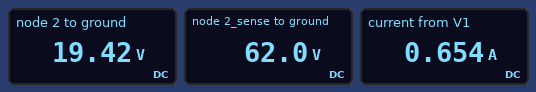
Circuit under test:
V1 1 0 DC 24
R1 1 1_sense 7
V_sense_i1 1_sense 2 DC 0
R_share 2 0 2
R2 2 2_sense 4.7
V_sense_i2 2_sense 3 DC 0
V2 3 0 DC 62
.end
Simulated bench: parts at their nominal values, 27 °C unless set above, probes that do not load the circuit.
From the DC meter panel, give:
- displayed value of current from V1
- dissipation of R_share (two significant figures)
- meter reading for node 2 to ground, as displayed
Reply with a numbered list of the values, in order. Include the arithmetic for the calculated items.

1. 0.654 A
2. (19.42 V)^2 / 2 Ω = 190 W
3. 19.42 V
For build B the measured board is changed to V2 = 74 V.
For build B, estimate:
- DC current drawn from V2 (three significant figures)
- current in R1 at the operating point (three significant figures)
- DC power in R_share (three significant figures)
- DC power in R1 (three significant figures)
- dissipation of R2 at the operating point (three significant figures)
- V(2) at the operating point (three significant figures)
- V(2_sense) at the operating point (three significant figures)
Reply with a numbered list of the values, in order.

1. 11.0 A
2. 227 mA
3. 251 W
4. 362 mW
5. 566 W
6. 22.4 V
7. 74.0 V
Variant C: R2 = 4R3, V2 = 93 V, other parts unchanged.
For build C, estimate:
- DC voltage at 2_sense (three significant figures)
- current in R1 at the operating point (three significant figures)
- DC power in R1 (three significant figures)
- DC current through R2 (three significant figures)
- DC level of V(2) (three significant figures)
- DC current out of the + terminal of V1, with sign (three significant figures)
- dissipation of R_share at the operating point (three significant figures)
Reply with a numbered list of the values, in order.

1. 93.0 V
2. 660 mA
3. 3.05 W
4. 15.0 A
5. 28.6 V
6. -660 mA
7. 410 W
